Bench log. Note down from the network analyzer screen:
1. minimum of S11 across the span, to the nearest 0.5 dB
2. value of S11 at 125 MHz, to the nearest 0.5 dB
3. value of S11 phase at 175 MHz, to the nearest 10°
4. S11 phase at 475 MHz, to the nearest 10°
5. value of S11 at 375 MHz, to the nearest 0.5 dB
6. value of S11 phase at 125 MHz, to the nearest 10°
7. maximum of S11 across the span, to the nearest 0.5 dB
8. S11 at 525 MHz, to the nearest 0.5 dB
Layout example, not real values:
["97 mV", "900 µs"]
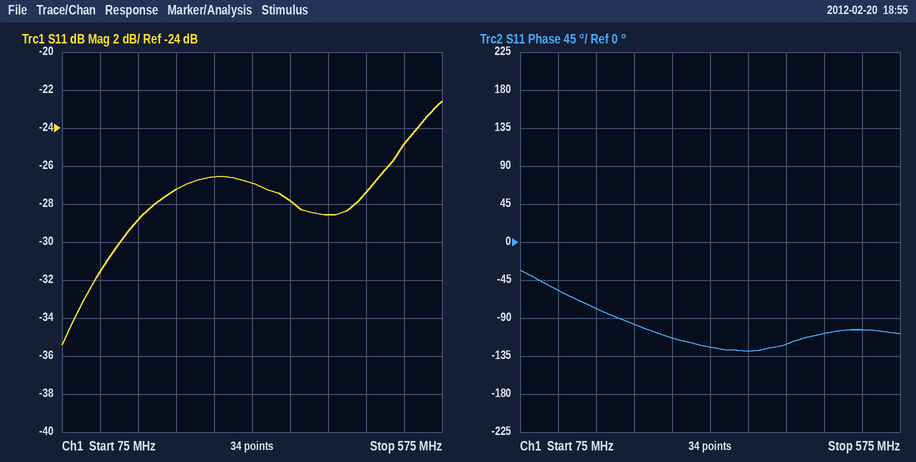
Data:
["-35.5 dB", "-31.5 dB", "-80°", "-110°", "-28.0 dB", "-60°", "-22.5 dB", "-25.0 dB"]
